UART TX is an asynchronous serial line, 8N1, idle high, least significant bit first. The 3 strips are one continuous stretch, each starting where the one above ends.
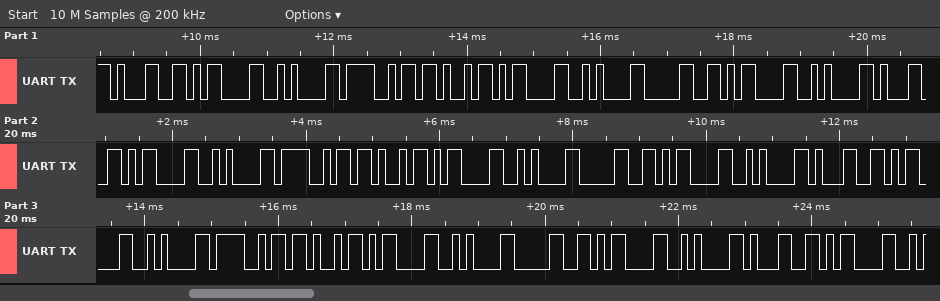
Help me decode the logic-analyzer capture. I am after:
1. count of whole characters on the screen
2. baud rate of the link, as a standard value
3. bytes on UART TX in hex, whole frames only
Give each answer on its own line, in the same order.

32
9600 baud
31 0D 0A 4F 4B 0D 0A 30 0D 0A 31 0D 0A 4F 4B 0D 0A 30 0D 0A 31 0D 0A 4F 4B 0D 0A 30 0D 0A 31 0D
